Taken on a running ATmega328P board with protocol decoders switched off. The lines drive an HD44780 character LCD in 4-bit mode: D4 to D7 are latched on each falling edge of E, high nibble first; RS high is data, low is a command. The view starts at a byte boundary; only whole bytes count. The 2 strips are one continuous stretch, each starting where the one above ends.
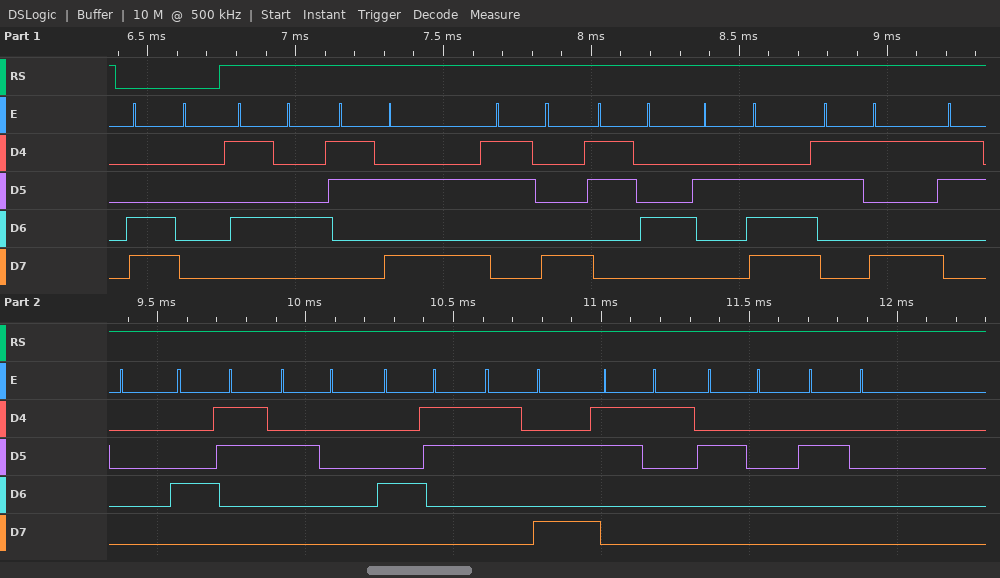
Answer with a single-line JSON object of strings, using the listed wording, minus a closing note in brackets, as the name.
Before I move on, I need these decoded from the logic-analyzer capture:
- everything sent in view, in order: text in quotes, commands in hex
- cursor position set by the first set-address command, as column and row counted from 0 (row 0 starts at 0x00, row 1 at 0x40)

{"everything sent in view, in order: text in quotes, commands in hex": "0xC0 \"T:84.90C C:1  \"", "cursor position set by the first set-address command, as column and row counted from 0": "column 0, row 1"}
